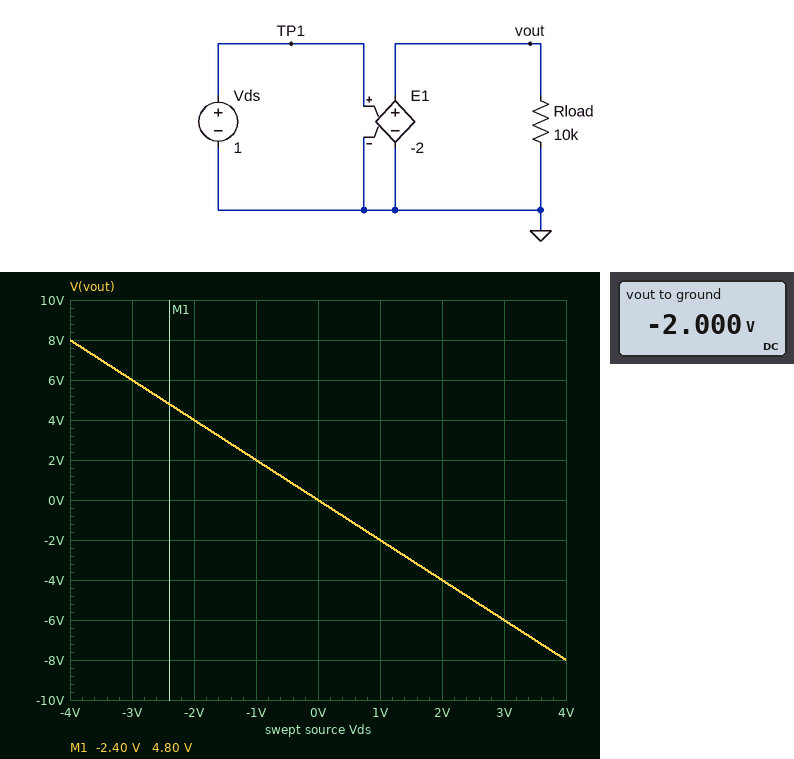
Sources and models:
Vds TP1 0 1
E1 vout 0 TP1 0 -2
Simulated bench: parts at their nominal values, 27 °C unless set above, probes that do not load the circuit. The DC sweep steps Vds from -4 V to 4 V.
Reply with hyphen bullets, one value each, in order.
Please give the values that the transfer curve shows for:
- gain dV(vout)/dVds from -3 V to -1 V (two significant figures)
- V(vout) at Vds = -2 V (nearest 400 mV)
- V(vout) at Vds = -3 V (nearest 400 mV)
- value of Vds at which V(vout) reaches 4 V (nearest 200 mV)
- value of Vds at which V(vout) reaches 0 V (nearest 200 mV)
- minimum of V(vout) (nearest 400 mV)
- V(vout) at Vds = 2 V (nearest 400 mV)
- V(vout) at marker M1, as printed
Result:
- -2.0 V/V
- 4.0 V
- 6.0 V
- -2.0 V
- 0 V
- -8.0 V
- -4.0 V
- 4.80 V
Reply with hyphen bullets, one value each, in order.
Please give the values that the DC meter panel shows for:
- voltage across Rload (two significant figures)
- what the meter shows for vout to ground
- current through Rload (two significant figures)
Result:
- 2.0 V
- -2.000 V
- 200 µA
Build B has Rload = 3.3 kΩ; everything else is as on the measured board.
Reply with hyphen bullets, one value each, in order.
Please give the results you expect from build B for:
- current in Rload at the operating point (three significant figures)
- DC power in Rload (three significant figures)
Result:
- 606 µA
- 1.21 mW
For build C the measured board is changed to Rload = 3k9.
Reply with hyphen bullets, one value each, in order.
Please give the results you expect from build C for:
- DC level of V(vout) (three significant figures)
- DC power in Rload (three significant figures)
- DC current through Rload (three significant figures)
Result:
- -2.00 V
- 1.03 mW
- 513 µA
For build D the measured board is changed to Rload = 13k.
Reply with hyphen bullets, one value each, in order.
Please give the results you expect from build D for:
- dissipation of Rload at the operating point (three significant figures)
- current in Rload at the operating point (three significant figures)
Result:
- 308 µW
- 154 µA
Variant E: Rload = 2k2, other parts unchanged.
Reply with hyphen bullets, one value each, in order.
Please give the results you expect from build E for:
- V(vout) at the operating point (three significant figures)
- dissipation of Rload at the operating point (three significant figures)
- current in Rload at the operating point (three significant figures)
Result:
- -2.00 V
- 1.82 mW
- 909 µA
